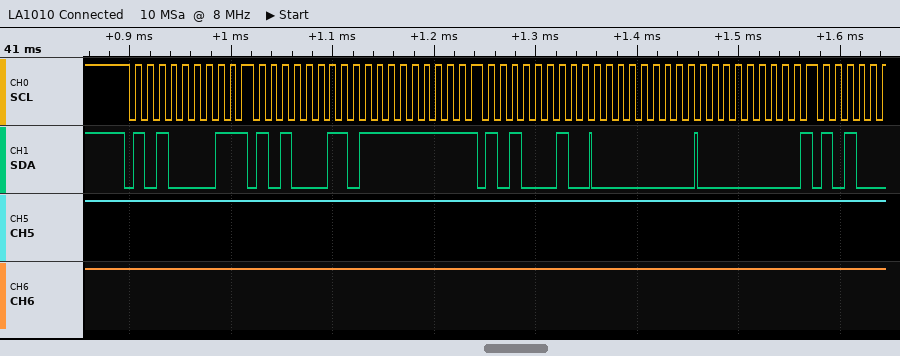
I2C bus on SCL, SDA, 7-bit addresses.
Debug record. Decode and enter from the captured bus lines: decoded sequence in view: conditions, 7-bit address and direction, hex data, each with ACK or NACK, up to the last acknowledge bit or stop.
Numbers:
start, address 50 read NACK, repeated start, address 51 read ACK, FF NACK, repeated start, address 51 write ACK, 00 ACK, 00 ACK
